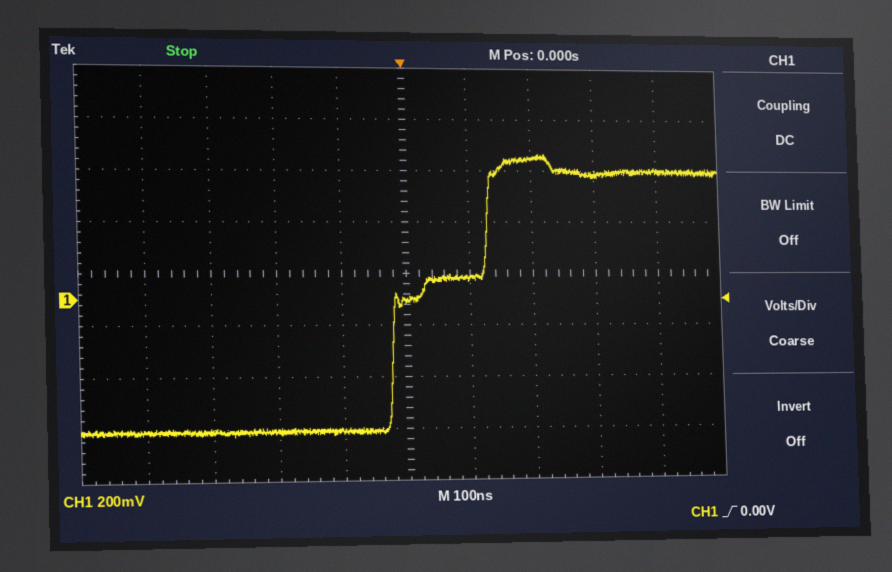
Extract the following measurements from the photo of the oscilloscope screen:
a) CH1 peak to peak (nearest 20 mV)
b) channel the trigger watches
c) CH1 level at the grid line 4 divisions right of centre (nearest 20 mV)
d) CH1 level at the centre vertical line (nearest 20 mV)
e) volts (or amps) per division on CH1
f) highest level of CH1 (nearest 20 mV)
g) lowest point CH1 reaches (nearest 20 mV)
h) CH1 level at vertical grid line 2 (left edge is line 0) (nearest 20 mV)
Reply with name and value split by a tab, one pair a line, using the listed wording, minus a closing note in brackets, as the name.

CH1 peak to peak	1.08 V
channel the trigger watches	CH1
CH1 level at the grid line 4 divisions right of centre	500 mV
CH1 level at the centre vertical line	0 mV
volts (or amps) per division on CH1	200 mV
highest level of CH1	560 mV
lowest point CH1 reaches	-520 mV
CH1 level at vertical grid line 2 (left edge is line 0)	-500 mV
